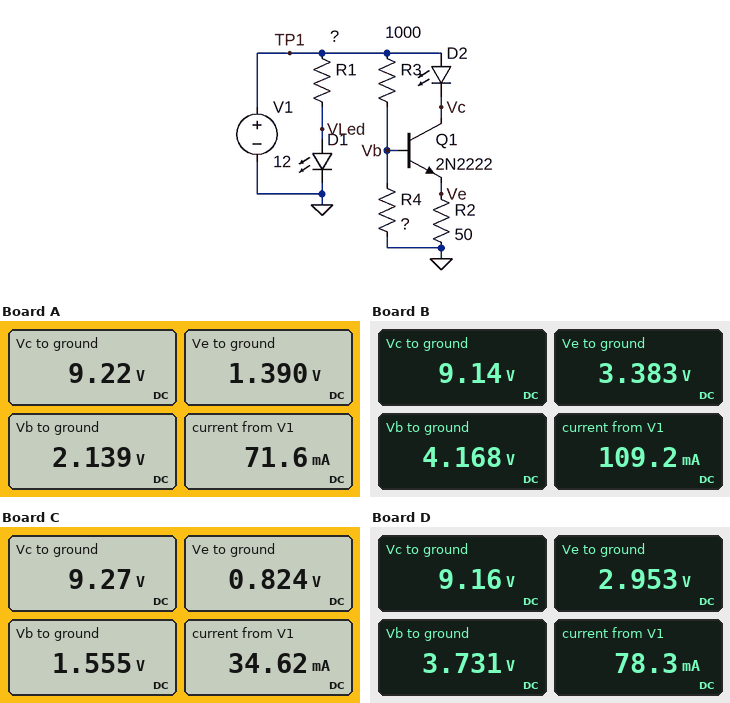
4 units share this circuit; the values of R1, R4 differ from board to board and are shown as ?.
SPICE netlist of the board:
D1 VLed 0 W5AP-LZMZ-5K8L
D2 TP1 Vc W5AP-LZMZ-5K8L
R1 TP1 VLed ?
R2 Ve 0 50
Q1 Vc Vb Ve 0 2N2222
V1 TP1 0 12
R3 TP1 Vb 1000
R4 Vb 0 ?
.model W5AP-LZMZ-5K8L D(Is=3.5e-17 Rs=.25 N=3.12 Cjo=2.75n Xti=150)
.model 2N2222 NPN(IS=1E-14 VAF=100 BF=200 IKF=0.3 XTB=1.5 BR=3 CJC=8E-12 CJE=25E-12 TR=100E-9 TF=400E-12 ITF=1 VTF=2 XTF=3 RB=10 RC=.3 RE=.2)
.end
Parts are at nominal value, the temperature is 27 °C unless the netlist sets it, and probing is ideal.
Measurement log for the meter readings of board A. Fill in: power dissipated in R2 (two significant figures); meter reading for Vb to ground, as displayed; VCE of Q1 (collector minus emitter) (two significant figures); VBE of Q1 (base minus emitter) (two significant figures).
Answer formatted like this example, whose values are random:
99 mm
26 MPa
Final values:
39 mW
2.139 V
7.8 V
750 mV
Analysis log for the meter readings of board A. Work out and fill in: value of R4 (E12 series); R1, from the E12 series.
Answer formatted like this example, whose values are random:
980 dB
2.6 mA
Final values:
220 Ω
270 Ω
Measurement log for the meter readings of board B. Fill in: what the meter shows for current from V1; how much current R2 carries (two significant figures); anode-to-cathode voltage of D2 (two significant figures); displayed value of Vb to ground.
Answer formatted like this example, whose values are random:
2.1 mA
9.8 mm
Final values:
109.2 mA
68 mA
2.9 V
4.168 V
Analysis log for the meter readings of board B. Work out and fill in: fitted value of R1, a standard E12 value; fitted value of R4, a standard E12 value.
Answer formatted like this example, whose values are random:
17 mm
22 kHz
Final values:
270 Ω
560 Ω
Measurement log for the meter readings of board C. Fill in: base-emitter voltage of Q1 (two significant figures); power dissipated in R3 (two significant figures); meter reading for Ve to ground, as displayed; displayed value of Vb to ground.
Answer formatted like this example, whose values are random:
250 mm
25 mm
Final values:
730 mV
110 mW
0.824 V
1.555 V
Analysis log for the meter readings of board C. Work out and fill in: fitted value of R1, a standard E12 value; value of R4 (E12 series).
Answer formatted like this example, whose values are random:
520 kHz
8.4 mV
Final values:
1.2 kΩ
150 Ω
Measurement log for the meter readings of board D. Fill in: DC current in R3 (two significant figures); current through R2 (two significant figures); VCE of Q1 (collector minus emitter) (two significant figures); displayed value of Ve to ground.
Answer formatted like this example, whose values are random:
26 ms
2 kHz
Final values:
8.3 mA
59 mA
6.2 V
2.953 V
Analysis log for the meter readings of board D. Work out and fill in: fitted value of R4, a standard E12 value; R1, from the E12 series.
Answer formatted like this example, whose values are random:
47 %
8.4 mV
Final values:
470 Ω
820 Ω
